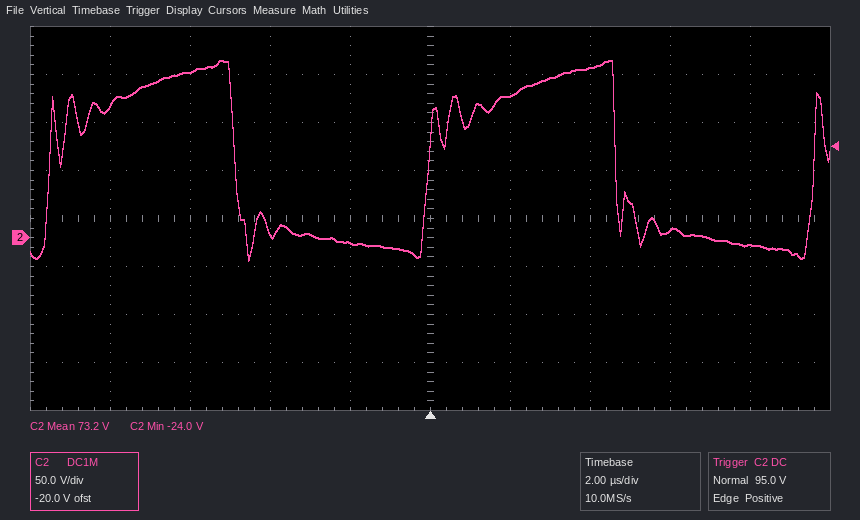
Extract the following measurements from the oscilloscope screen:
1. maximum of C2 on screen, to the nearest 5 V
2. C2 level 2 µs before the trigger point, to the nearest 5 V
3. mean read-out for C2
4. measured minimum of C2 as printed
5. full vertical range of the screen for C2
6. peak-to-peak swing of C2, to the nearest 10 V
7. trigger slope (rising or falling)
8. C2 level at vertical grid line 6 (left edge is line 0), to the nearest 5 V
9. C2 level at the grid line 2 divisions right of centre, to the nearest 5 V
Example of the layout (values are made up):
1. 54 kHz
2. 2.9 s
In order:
1. 185 V
2. -5 V
3. 73.2 V
4. -24.0 V
5. 400 V
6. 210 V
7. rising
8. 150 V
9. 175 V
